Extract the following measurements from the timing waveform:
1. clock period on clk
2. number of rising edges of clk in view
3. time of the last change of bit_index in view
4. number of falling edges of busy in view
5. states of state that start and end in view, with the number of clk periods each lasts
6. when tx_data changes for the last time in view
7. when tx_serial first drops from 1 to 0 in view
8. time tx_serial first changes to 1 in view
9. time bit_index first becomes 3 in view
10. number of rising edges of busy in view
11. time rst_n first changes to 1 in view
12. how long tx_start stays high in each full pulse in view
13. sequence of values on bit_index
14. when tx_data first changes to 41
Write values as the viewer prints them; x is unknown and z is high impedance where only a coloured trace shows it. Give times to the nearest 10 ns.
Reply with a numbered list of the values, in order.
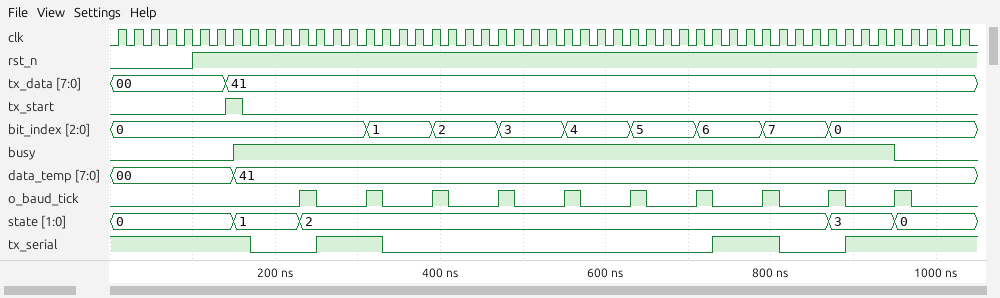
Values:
1. 20 ns
2. 52
3. 870 ns
4. 1
5. 1: 4, 2: 32, 3: 4
6. 140 ns
7. 170 ns
8. 250 ns
9. 470 ns
10. 1
11. 100 ns
12. 20 ns
13. 0, 1, 2, 3, 4, 5, 6, 7, 0
14. 140 ns
